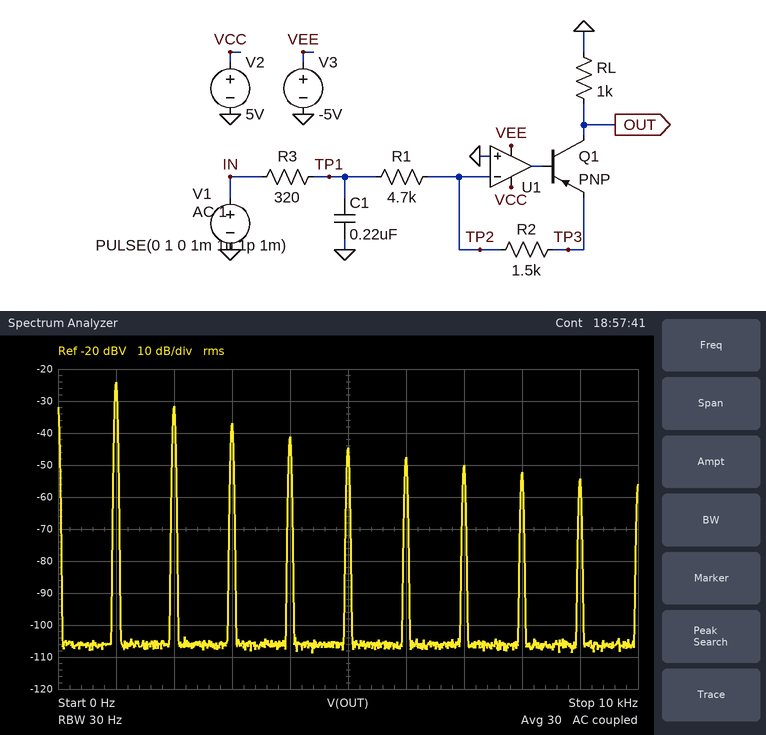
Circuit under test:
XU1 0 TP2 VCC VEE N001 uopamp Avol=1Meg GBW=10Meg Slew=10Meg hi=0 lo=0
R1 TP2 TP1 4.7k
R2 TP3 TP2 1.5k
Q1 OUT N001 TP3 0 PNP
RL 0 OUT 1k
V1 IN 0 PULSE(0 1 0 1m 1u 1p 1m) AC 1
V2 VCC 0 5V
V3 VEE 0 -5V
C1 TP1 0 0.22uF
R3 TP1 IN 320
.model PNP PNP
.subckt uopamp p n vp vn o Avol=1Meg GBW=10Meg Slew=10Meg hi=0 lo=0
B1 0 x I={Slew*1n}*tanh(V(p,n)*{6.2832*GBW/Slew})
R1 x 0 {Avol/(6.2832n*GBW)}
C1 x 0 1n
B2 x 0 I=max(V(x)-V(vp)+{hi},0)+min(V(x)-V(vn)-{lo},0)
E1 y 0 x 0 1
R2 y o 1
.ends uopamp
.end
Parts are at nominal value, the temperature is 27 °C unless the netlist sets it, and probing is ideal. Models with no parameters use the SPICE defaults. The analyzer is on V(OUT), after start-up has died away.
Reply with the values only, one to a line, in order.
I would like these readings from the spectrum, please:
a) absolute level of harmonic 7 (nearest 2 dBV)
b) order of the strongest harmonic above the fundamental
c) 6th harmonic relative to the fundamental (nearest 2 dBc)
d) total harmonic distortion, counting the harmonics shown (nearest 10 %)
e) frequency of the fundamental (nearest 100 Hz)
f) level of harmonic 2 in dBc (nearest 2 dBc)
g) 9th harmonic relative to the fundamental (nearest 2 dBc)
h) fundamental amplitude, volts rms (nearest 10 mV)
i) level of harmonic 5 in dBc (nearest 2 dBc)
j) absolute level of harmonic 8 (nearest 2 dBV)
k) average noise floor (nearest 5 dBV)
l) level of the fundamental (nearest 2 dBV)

-50 dBV
2
-24 dBc
50 %
1.0 kHz
-8 dBc
-30 dBc
60 mV
-20 dBc
-52 dBV
-105 dBV
-24 dBV
